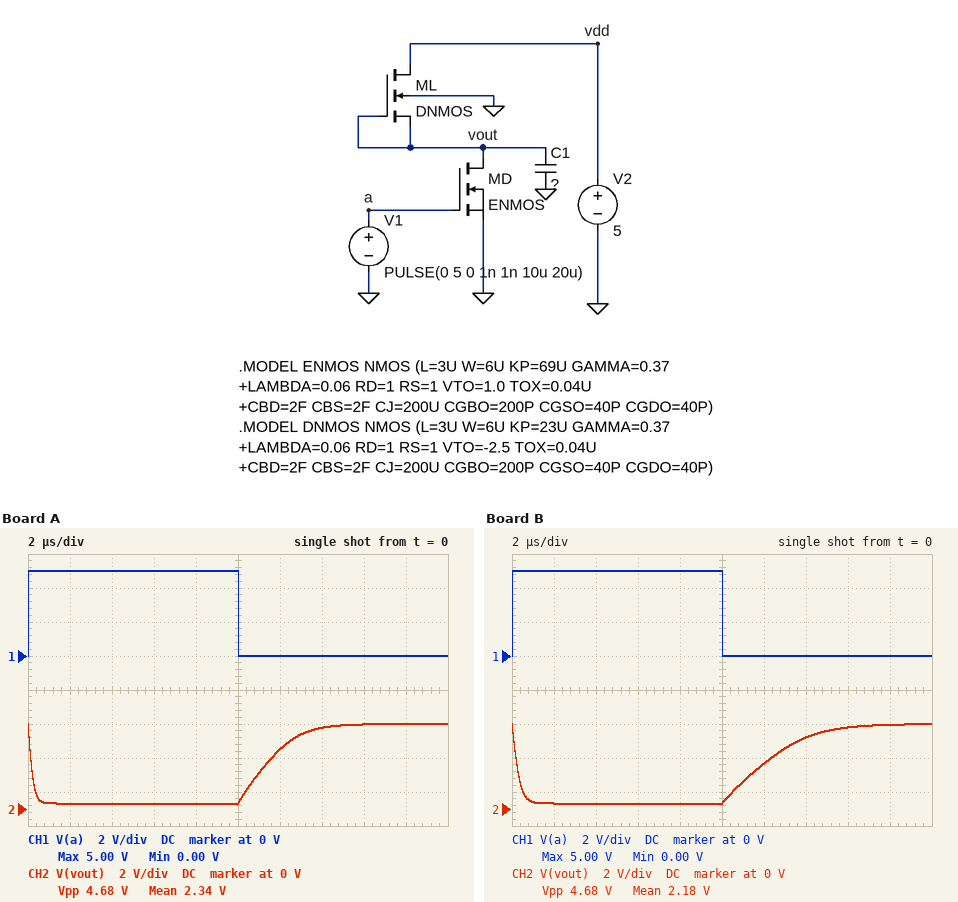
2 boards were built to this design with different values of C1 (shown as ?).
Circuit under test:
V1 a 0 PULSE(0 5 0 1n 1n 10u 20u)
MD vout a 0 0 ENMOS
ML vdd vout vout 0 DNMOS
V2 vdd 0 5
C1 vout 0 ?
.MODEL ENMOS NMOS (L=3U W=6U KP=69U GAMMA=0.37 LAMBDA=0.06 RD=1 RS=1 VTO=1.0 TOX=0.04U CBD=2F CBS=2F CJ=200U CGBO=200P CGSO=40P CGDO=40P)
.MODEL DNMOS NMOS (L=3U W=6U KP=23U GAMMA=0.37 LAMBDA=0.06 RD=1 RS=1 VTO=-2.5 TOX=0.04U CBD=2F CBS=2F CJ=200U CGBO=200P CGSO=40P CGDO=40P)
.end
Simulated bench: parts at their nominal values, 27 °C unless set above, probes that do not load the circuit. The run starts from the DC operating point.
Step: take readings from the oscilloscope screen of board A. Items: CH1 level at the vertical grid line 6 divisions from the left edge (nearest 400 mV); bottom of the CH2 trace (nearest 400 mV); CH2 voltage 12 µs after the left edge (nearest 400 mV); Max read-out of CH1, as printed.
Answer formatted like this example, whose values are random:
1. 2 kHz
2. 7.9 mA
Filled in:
1. 0 V
2. 400 mV
3. 3.6 V
4. 5.00 V
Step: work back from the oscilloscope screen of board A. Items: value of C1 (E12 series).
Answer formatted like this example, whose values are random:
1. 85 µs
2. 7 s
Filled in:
1. 82 pF
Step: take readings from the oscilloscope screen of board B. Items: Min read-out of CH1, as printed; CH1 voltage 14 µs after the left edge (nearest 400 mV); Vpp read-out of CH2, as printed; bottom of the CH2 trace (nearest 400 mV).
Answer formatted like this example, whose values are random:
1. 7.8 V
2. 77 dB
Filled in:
1. 0.00 V
2. 0 V
3. 4.68 V
4. 400 mV
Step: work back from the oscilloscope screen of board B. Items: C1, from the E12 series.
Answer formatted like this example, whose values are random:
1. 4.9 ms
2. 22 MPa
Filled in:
1. 120 pF
